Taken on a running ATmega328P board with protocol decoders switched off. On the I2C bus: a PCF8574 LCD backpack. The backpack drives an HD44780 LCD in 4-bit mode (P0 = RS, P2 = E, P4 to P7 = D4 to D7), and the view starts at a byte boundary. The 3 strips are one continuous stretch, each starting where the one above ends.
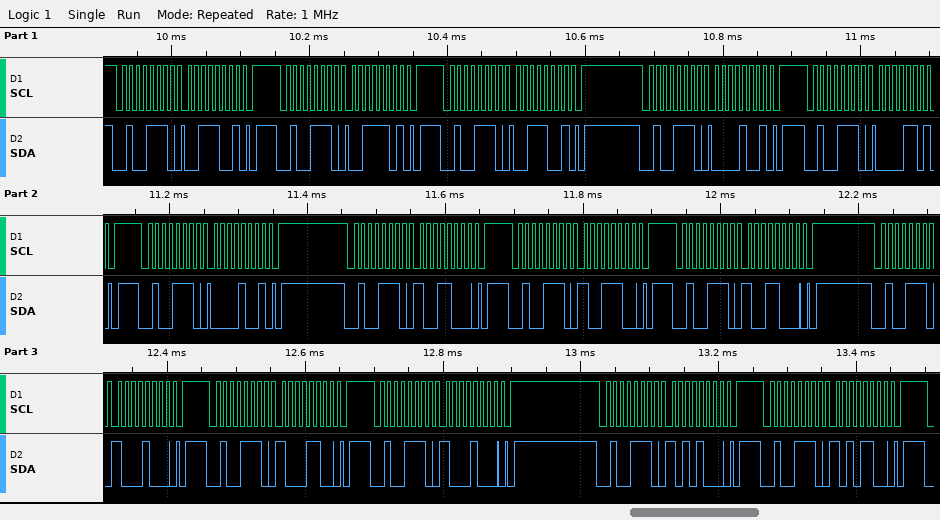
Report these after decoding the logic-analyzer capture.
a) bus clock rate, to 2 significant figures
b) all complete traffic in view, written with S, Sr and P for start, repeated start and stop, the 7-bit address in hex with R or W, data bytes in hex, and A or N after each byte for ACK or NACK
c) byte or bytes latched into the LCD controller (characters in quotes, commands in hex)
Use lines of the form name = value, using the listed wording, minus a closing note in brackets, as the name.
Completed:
bus clock rate, to 2 significant figures = 100 kHz
all complete traffic in view, written with S, Sr and P for start, repeated start and stop, the 7-bit address in hex with R or W, data bytes in hex, and A or N after each byte for ACK or NACK = S 27W A 39 A P S 27W A 3D A P S 27W A 39 A P S 27W A 09 A P S 27W A 0D A P S 27W A 09 A P S 27W A 98 A P S 27W A 9C A P S 27W A 98 A P S 27W A 88 A P S 27W A 8C A P S 27W A 88 A P S 27W A A8 A P S 27W A AC A P
byte or bytes latched into the LCD controller = '0' 0x98
